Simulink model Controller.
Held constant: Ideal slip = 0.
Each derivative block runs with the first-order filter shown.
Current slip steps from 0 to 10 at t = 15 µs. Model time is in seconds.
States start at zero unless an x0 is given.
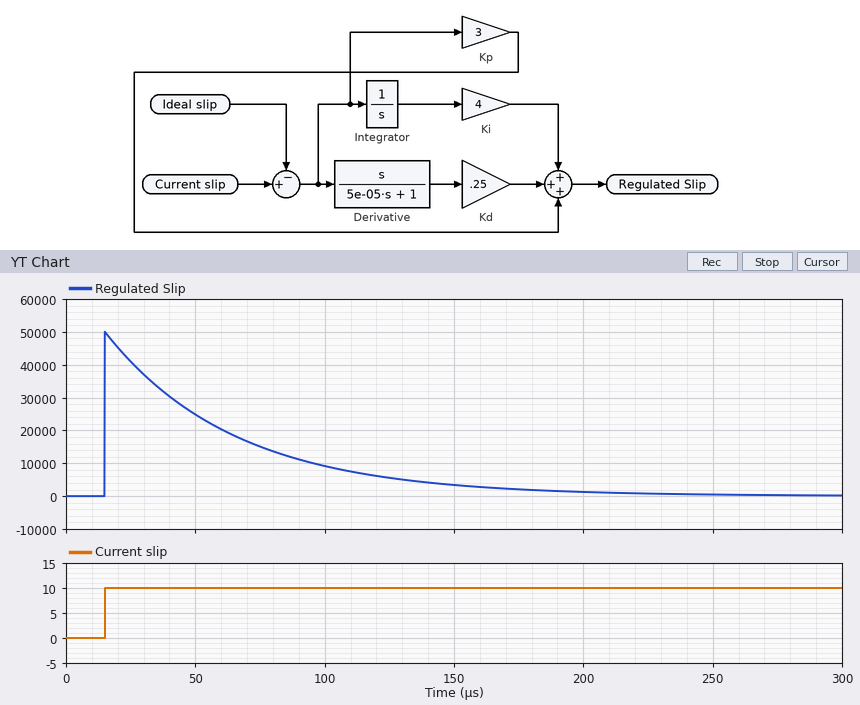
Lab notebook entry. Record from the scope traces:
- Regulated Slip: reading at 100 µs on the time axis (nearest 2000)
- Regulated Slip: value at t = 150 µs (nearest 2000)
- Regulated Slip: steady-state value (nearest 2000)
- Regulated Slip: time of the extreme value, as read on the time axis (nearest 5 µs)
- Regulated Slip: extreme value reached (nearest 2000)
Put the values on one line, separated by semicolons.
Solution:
10000; 4000; 0; 15 µs; 50000
